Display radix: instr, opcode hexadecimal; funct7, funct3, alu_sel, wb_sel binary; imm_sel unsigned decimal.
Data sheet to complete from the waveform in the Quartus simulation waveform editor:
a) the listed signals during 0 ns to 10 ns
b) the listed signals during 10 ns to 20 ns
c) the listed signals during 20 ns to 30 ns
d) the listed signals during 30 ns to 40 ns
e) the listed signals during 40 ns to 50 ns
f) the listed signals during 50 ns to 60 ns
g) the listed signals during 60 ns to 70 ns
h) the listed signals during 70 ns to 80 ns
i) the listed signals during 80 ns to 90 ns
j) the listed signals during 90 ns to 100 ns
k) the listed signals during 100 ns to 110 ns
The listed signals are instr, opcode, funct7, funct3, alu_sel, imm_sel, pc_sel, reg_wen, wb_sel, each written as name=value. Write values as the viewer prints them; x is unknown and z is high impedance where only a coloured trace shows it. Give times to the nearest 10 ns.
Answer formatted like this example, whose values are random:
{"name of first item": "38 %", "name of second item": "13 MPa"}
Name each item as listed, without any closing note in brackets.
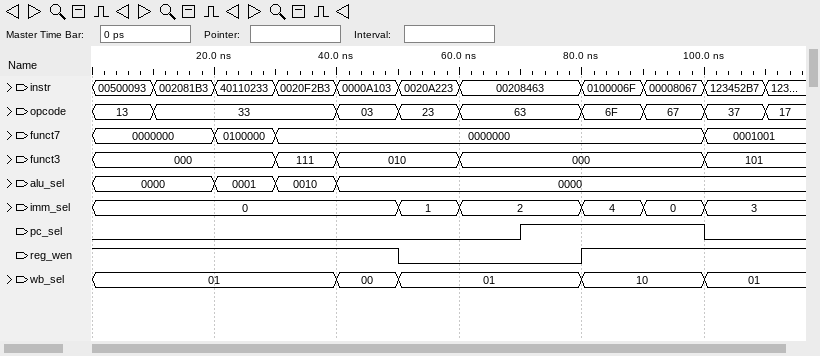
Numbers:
{"the listed signals during 0 ns to 10 ns": "instr=00500093, opcode=13, funct7=0000000, funct3=000, alu_sel=0000, imm_sel=0, pc_sel=0, reg_wen=1, wb_sel=01", "the listed signals during 10 ns to 20 ns": "instr=002081B3, opcode=33, funct7=0000000, funct3=000, alu_sel=0000, imm_sel=0, pc_sel=0, reg_wen=1, wb_sel=01", "the listed signals during 20 ns to 30 ns": "instr=40110233, opcode=33, funct7=0100000, funct3=000, alu_sel=0001, imm_sel=0, pc_sel=0, reg_wen=1, wb_sel=01", "the listed signals during 30 ns to 40 ns": "instr=0020F2B3, opcode=33, funct7=0000000, funct3=111, alu_sel=0010, imm_sel=0, pc_sel=0, reg_wen=1, wb_sel=01", "the listed signals during 40 ns to 50 ns": "instr=0000A103, opcode=03, funct7=0000000, funct3=010, alu_sel=0000, imm_sel=0, pc_sel=0, reg_wen=1, wb_sel=00", "the listed signals during 50 ns to 60 ns": "instr=0020A223, opcode=23, funct7=0000000, funct3=010, alu_sel=0000, imm_sel=1, pc_sel=0, reg_wen=0, wb_sel=01", "the listed signals during 60 ns to 70 ns": "instr=00208463, opcode=63, funct7=0000000, funct3=000, alu_sel=0000, imm_sel=2, pc_sel=0, reg_wen=0, wb_sel=01", "the listed signals during 70 ns to 80 ns": "instr=00208463, opcode=63, funct7=0000000, funct3=000, alu_sel=0000, imm_sel=2, pc_sel=1, reg_wen=0, wb_sel=01", "the listed signals during 80 ns to 90 ns": "instr=0100006F, opcode=6F, funct7=0000000, funct3=000, alu_sel=0000, imm_sel=4, pc_sel=1, reg_wen=1, wb_sel=10", "the listed signals during 90 ns to 100 ns": "instr=00008067, opcode=67, funct7=0000000, funct3=000, alu_sel=0000, imm_sel=0, pc_sel=1, reg_wen=1, wb_sel=10", "the listed signals during 100 ns to 110 ns": "instr=123452B7, opcode=37, funct7=0001001, funct3=101, alu_sel=0000, imm_sel=3, pc_sel=0, reg_wen=1, wb_sel=01"}
